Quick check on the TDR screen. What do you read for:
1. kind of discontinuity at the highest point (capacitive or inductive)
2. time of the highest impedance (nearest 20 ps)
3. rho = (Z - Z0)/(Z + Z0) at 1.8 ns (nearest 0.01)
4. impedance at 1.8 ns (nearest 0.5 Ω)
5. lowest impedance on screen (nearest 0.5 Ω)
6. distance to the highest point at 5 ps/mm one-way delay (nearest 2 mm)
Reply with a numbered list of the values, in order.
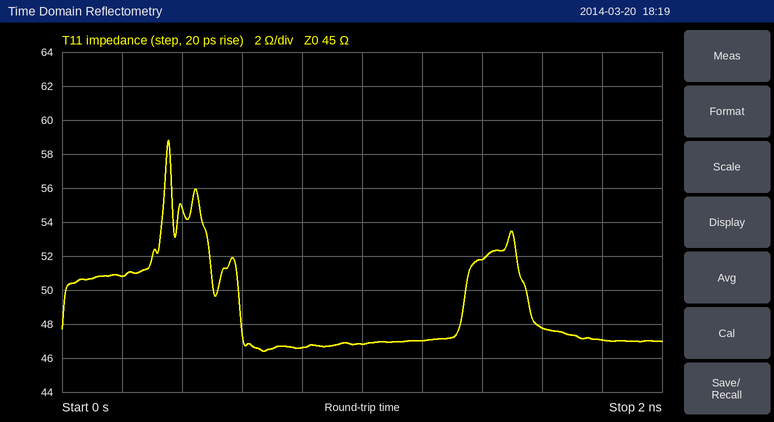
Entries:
1. inductive
2. 360 ps
3. +0.02
4. 47.0 Ω
5. 46.5 Ω
6. 36 mm
